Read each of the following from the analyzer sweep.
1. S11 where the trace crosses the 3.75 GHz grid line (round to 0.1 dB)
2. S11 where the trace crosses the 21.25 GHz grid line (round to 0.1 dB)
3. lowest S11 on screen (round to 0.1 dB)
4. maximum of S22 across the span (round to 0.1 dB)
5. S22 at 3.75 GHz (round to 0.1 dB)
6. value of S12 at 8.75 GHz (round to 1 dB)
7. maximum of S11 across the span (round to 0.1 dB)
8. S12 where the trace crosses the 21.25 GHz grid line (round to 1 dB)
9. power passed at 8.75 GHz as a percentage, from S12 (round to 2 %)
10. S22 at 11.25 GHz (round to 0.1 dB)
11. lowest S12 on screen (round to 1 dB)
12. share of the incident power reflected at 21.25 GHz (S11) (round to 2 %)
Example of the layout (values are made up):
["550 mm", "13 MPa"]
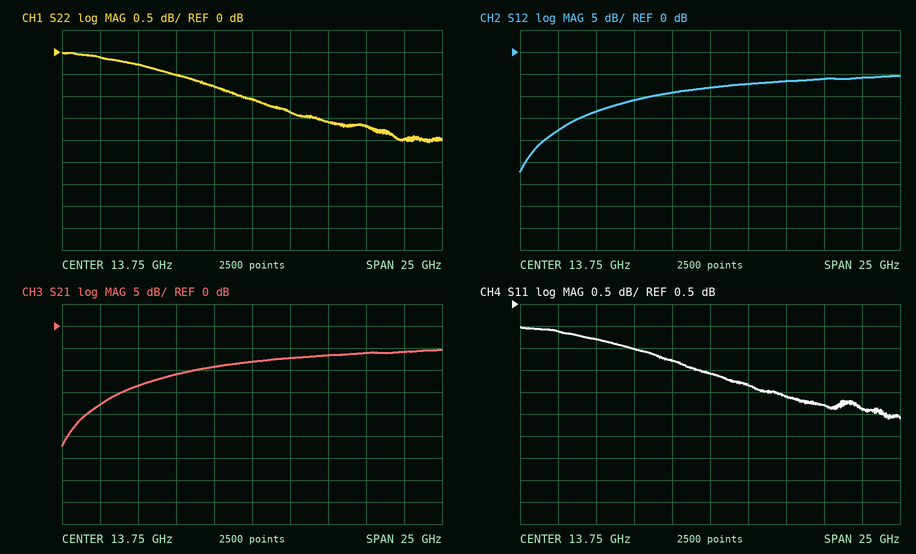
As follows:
["-0.1 dB", "-1.8 dB", "-2.1 dB", "0.0 dB", "-0.1 dB", "-11 dB", "0.0 dB", "-6 dB", "8 %", "-0.8 dB", "-27 dB", "66 %"]
